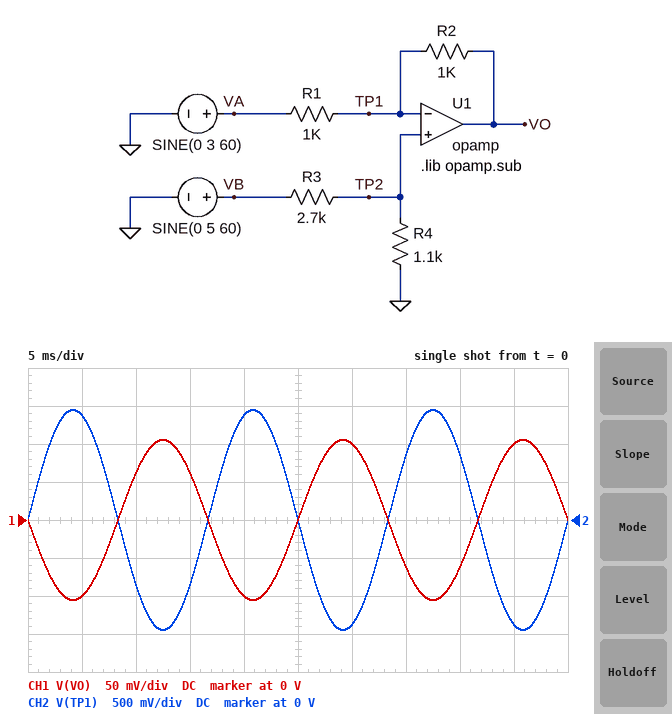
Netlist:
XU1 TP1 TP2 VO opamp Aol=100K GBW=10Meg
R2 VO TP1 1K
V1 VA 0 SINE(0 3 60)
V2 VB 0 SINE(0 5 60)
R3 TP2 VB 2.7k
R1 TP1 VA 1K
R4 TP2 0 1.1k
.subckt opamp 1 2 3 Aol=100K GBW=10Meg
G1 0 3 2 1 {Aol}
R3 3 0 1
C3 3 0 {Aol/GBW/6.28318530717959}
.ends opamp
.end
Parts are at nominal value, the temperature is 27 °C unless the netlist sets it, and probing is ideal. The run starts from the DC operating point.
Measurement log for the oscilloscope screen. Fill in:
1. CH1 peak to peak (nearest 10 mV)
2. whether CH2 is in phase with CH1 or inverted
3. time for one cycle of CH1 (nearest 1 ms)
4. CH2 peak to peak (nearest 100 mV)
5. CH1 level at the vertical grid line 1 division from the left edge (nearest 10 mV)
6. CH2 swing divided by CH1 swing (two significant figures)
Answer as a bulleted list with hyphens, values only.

- 210 mV
- inverted
- 17 ms
- 2.9 V
- -100 mV
- 14
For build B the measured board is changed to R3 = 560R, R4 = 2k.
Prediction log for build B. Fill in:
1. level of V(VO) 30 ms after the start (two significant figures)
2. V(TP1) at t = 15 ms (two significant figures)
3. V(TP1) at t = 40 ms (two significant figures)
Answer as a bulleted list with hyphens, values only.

- -4.6 V
- -2.3 V
- 2.3 V
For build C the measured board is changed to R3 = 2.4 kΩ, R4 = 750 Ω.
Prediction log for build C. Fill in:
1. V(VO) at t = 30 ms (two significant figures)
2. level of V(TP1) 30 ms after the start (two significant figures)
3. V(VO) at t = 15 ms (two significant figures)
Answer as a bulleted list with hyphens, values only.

- 590 mV
- -1.1 V
- 360 mV
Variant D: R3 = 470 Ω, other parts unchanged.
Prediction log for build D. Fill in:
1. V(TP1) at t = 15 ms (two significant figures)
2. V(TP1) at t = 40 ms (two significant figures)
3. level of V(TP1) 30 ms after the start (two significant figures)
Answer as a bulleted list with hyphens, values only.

- -2.1 V
- 2.1 V
- -3.3 V
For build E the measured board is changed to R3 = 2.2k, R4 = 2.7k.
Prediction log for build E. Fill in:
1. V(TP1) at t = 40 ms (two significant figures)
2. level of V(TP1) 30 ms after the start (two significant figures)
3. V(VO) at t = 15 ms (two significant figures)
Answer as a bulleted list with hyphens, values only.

- 1.6 V
- -2.6 V
- -1.5 V
